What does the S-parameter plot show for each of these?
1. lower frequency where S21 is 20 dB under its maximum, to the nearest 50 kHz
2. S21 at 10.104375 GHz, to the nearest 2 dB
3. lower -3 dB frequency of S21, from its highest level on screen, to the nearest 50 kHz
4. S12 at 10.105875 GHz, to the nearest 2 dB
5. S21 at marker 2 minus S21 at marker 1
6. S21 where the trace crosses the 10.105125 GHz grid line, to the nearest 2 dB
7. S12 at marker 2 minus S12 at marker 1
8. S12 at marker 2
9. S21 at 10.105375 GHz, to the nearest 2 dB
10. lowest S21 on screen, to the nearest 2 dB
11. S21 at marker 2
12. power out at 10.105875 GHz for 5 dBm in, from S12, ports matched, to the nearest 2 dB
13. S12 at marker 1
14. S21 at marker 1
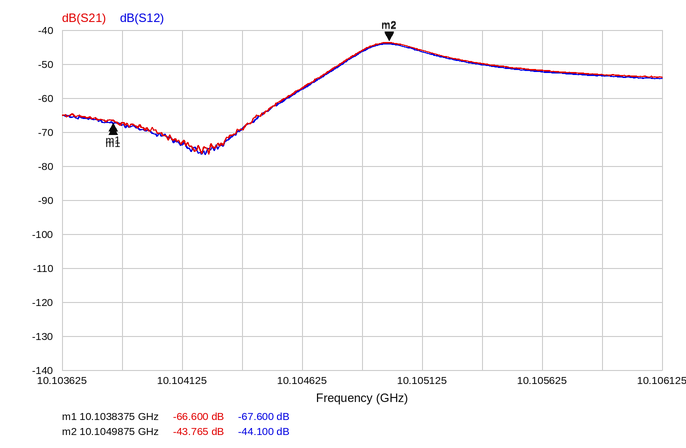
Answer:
10.10450 GHz
-70 dB
10.10485 GHz
-54 dB
22.835 dB
-46 dB
23.500 dB
-44.100 dB
-50 dB
-76 dB
-43.765 dB
-48 dBm
-67.600 dB
-66.600 dB
